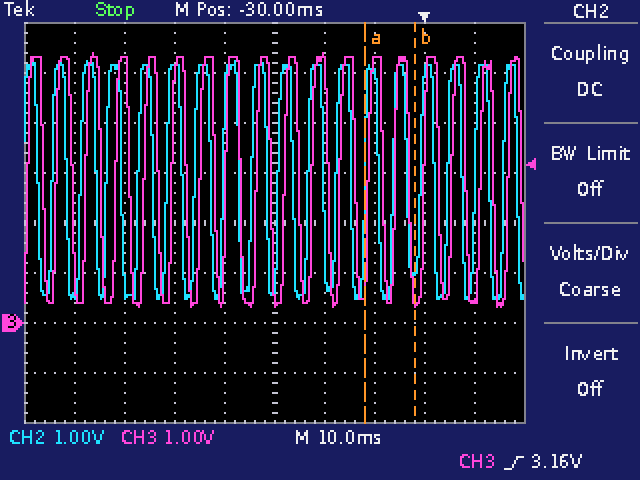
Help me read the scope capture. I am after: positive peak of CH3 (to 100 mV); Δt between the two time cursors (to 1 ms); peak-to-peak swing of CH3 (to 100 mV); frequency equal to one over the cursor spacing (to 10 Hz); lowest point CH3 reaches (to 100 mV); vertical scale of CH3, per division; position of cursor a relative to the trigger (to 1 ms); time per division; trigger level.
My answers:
5.4 V
10 ms
5.1 V
100 Hz
300 mV
1 V
-12 ms
10 ms
3.16 V
